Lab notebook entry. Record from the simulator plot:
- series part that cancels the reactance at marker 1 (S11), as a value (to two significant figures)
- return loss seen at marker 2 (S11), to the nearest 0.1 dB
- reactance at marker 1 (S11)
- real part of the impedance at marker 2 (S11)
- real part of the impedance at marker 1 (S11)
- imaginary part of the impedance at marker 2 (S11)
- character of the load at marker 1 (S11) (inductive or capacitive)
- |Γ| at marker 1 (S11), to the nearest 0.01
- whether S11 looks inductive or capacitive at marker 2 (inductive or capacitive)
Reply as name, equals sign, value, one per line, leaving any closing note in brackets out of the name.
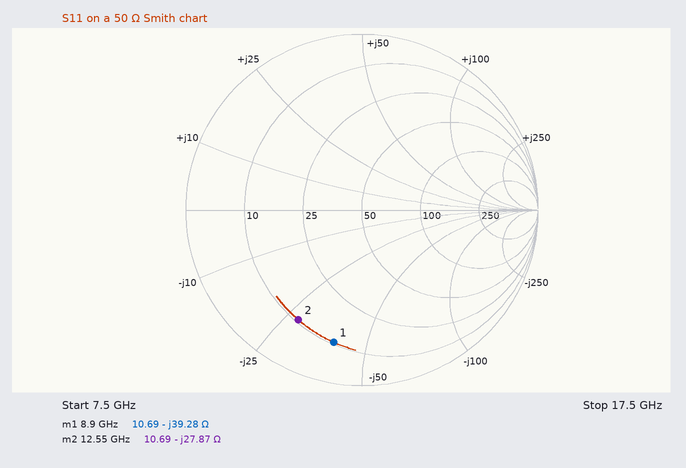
series part that cancels the reactance at marker 1 (S11), as a value = 700 pH
return loss seen at marker 2 (S11), to the nearest 0.1 dB = 2.8 dB
reactance at marker 1 = -39.28 Ω
real part of the impedance at marker 2 = 10.69 Ω
real part of the impedance at marker 1 = 10.69 Ω
imaginary part of the impedance at marker 2 = -27.87 Ω
character of the load at marker 1 (S11) = capacitive
|Γ| at marker 1 (S11), to the nearest 0.01 = 0.77
whether S11 looks inductive or capacitive at marker 2 = capacitive
